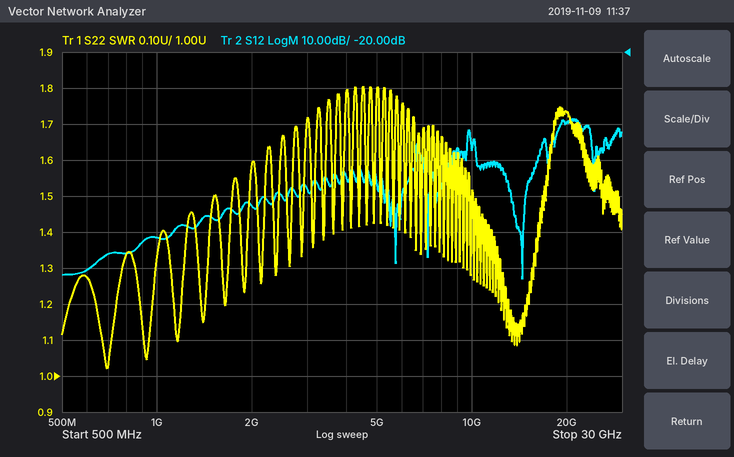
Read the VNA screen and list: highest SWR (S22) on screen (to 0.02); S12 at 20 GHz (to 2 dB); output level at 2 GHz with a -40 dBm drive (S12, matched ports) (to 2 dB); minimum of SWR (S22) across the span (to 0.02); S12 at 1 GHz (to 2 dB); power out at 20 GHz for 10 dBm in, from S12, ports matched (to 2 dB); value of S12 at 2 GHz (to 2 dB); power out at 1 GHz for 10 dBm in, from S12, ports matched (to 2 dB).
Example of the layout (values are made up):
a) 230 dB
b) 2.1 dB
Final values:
a) 1.80
b) -40 dB
c) -102 dBm
d) 1.02
e) -72 dB
f) -30 dBm
g) -62 dB
h) -62 dBm
